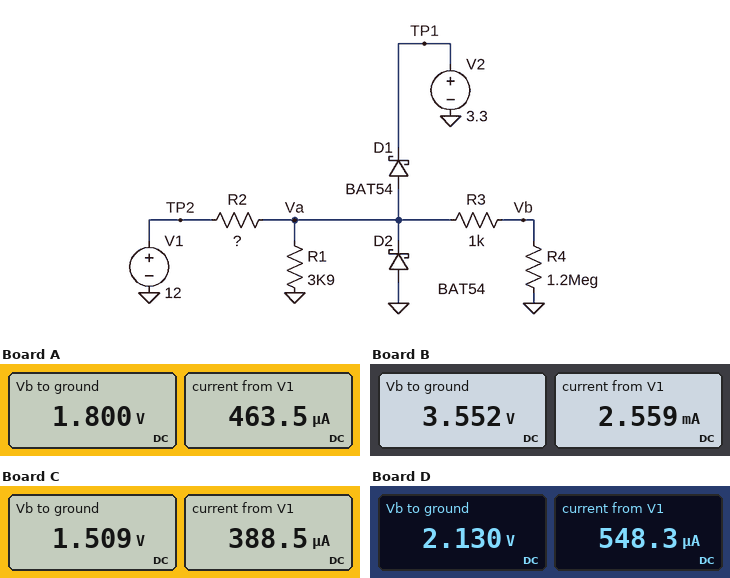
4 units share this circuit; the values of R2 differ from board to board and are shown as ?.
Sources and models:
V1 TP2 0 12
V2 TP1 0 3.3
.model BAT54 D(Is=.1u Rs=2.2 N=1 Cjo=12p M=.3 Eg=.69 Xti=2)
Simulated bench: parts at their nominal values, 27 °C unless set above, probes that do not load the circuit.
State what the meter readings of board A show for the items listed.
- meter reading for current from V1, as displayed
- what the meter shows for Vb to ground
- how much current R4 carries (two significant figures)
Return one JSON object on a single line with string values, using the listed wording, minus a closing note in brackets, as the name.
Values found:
{"meter reading for current from V1, as displayed": "463.5 µA", "what the meter shows for Vb to ground": "1.800 V", "how much current R4 carries": "1.5 µA"}
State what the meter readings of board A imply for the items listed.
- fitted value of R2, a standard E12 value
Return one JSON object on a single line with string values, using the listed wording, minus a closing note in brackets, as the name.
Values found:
{"fitted value of R2, a standard E12 value": "22 kΩ"}
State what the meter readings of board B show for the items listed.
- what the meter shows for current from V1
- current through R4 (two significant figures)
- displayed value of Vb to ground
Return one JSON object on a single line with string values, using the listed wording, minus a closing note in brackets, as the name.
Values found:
{"what the meter shows for current from V1": "2.559 mA", "current through R4": "3.0 µA", "displayed value of Vb to ground": "3.552 V"}
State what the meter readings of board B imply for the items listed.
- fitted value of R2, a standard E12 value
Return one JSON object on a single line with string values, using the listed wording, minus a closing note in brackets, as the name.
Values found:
{"fitted value of R2, a standard E12 value": "3.3 kΩ"}
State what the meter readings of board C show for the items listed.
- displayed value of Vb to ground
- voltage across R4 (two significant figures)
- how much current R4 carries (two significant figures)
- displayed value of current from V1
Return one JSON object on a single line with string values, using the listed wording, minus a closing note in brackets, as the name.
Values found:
{"displayed value of Vb to ground": "1.509 V", "voltage across R4": "1.5 V", "how much current R4 carries": "1.3 µA", "displayed value of current from V1": "388.5 µA"}
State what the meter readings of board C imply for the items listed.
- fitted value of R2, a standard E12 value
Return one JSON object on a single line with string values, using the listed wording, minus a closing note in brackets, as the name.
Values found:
{"fitted value of R2, a standard E12 value": "27 kΩ"}
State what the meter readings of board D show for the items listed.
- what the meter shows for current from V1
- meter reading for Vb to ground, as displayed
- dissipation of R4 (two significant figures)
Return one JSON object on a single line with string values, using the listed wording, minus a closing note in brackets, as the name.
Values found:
{"what the meter shows for current from V1": "548.3 µA", "meter reading for Vb to ground, as displayed": "2.130 V", "dissipation of R4": "3.8 µW"}
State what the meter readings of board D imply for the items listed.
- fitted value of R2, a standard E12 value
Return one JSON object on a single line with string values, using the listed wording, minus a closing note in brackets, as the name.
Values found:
{"fitted value of R2, a standard E12 value": "18 kΩ"}
